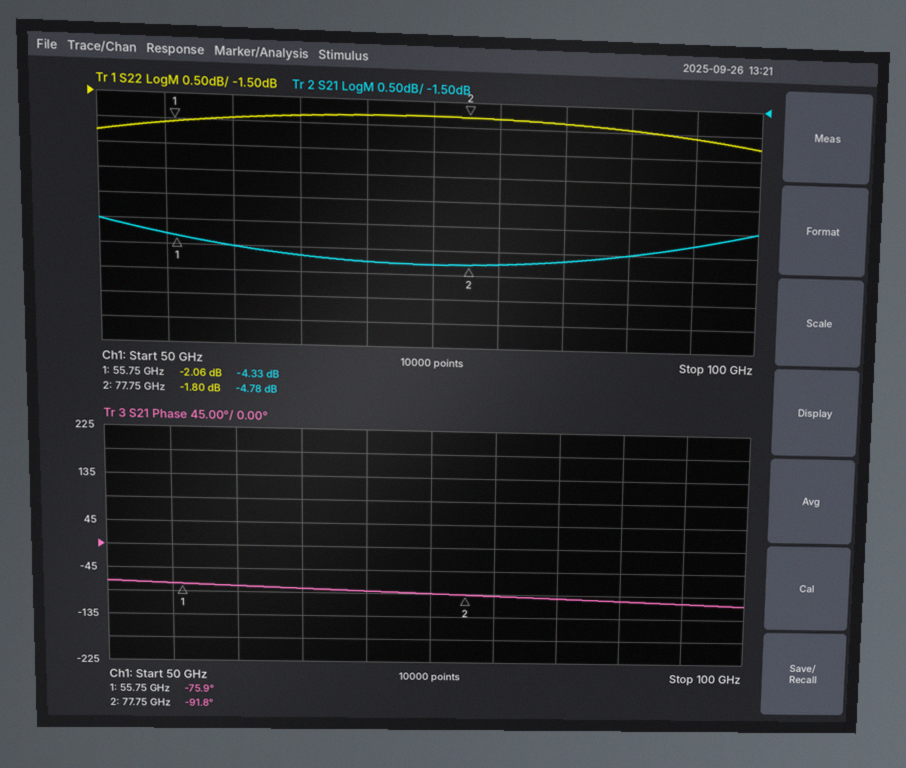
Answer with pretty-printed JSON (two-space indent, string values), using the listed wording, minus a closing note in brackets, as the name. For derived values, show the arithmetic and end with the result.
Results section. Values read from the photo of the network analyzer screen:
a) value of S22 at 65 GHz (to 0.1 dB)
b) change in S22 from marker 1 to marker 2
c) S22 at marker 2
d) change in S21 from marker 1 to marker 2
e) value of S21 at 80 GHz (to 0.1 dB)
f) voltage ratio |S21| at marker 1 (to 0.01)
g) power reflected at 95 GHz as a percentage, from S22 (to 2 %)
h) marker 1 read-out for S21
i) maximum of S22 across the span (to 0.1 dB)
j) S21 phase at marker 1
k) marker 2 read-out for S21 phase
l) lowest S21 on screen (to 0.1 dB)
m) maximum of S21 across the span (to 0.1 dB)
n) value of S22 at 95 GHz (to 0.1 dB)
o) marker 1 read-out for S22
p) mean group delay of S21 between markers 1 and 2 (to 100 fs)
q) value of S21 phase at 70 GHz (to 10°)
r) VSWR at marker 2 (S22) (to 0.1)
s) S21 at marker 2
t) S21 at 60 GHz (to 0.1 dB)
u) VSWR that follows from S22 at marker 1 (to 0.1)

{
  "value of S22 at 65 GHz": "-1.9 dB",
  "change in S22 from marker 1 to marker 2": "-1.8 − (-2.06) = 0.26 dB",
  "S22 at marker 2": "-1.80 dB",
  "change in S21 from marker 1 to marker 2": "-4.78 − (-4.33) = -0.45 dB",
  "value of S21 at 80 GHz": "-4.8 dB",
  "voltage ratio |S21| at marker 1": "10^(-4.33/20) ≈ 0.61",
  "power reflected at 95 GHz as a percentage, from S22": "10^(-2.1/10) ≈ 62 %",
  "marker 1 read-out for S21": "-4.33 dB",
  "maximum of S22 across the span": "-1.8 dB",
  "S21 phase at marker 1": "-75.9°",
  "marker 2 read-out for S21 phase": "-91.8°",
  "lowest S21 on screen": "-4.8 dB",
  "maximum of S21 across the span": "-4.0 dB",
  "value of S22 at 95 GHz": "-2.1 dB",
  "marker 1 read-out for S22": "-2.06 dB",
  "mean group delay of S21 between markers 1 and 2": "−(-91.8° − (-75.9°))/(360° × 22 GHz) ≈ 2.0 ps",
  "value of S21 phase at 70 GHz": "-90°",
  "VSWR at marker 2 (S22)": "(1 + 0.8128)/(1 − 0.8128) ≈ 9.7",
  "S21 at marker 2": "-4.78 dB",
  "S21 at 60 GHz": "-4.5 dB",
  "VSWR that follows from S22 at marker 1": "(1 + 0.7889)/(1 − 0.7889) ≈ 8.5"
}
